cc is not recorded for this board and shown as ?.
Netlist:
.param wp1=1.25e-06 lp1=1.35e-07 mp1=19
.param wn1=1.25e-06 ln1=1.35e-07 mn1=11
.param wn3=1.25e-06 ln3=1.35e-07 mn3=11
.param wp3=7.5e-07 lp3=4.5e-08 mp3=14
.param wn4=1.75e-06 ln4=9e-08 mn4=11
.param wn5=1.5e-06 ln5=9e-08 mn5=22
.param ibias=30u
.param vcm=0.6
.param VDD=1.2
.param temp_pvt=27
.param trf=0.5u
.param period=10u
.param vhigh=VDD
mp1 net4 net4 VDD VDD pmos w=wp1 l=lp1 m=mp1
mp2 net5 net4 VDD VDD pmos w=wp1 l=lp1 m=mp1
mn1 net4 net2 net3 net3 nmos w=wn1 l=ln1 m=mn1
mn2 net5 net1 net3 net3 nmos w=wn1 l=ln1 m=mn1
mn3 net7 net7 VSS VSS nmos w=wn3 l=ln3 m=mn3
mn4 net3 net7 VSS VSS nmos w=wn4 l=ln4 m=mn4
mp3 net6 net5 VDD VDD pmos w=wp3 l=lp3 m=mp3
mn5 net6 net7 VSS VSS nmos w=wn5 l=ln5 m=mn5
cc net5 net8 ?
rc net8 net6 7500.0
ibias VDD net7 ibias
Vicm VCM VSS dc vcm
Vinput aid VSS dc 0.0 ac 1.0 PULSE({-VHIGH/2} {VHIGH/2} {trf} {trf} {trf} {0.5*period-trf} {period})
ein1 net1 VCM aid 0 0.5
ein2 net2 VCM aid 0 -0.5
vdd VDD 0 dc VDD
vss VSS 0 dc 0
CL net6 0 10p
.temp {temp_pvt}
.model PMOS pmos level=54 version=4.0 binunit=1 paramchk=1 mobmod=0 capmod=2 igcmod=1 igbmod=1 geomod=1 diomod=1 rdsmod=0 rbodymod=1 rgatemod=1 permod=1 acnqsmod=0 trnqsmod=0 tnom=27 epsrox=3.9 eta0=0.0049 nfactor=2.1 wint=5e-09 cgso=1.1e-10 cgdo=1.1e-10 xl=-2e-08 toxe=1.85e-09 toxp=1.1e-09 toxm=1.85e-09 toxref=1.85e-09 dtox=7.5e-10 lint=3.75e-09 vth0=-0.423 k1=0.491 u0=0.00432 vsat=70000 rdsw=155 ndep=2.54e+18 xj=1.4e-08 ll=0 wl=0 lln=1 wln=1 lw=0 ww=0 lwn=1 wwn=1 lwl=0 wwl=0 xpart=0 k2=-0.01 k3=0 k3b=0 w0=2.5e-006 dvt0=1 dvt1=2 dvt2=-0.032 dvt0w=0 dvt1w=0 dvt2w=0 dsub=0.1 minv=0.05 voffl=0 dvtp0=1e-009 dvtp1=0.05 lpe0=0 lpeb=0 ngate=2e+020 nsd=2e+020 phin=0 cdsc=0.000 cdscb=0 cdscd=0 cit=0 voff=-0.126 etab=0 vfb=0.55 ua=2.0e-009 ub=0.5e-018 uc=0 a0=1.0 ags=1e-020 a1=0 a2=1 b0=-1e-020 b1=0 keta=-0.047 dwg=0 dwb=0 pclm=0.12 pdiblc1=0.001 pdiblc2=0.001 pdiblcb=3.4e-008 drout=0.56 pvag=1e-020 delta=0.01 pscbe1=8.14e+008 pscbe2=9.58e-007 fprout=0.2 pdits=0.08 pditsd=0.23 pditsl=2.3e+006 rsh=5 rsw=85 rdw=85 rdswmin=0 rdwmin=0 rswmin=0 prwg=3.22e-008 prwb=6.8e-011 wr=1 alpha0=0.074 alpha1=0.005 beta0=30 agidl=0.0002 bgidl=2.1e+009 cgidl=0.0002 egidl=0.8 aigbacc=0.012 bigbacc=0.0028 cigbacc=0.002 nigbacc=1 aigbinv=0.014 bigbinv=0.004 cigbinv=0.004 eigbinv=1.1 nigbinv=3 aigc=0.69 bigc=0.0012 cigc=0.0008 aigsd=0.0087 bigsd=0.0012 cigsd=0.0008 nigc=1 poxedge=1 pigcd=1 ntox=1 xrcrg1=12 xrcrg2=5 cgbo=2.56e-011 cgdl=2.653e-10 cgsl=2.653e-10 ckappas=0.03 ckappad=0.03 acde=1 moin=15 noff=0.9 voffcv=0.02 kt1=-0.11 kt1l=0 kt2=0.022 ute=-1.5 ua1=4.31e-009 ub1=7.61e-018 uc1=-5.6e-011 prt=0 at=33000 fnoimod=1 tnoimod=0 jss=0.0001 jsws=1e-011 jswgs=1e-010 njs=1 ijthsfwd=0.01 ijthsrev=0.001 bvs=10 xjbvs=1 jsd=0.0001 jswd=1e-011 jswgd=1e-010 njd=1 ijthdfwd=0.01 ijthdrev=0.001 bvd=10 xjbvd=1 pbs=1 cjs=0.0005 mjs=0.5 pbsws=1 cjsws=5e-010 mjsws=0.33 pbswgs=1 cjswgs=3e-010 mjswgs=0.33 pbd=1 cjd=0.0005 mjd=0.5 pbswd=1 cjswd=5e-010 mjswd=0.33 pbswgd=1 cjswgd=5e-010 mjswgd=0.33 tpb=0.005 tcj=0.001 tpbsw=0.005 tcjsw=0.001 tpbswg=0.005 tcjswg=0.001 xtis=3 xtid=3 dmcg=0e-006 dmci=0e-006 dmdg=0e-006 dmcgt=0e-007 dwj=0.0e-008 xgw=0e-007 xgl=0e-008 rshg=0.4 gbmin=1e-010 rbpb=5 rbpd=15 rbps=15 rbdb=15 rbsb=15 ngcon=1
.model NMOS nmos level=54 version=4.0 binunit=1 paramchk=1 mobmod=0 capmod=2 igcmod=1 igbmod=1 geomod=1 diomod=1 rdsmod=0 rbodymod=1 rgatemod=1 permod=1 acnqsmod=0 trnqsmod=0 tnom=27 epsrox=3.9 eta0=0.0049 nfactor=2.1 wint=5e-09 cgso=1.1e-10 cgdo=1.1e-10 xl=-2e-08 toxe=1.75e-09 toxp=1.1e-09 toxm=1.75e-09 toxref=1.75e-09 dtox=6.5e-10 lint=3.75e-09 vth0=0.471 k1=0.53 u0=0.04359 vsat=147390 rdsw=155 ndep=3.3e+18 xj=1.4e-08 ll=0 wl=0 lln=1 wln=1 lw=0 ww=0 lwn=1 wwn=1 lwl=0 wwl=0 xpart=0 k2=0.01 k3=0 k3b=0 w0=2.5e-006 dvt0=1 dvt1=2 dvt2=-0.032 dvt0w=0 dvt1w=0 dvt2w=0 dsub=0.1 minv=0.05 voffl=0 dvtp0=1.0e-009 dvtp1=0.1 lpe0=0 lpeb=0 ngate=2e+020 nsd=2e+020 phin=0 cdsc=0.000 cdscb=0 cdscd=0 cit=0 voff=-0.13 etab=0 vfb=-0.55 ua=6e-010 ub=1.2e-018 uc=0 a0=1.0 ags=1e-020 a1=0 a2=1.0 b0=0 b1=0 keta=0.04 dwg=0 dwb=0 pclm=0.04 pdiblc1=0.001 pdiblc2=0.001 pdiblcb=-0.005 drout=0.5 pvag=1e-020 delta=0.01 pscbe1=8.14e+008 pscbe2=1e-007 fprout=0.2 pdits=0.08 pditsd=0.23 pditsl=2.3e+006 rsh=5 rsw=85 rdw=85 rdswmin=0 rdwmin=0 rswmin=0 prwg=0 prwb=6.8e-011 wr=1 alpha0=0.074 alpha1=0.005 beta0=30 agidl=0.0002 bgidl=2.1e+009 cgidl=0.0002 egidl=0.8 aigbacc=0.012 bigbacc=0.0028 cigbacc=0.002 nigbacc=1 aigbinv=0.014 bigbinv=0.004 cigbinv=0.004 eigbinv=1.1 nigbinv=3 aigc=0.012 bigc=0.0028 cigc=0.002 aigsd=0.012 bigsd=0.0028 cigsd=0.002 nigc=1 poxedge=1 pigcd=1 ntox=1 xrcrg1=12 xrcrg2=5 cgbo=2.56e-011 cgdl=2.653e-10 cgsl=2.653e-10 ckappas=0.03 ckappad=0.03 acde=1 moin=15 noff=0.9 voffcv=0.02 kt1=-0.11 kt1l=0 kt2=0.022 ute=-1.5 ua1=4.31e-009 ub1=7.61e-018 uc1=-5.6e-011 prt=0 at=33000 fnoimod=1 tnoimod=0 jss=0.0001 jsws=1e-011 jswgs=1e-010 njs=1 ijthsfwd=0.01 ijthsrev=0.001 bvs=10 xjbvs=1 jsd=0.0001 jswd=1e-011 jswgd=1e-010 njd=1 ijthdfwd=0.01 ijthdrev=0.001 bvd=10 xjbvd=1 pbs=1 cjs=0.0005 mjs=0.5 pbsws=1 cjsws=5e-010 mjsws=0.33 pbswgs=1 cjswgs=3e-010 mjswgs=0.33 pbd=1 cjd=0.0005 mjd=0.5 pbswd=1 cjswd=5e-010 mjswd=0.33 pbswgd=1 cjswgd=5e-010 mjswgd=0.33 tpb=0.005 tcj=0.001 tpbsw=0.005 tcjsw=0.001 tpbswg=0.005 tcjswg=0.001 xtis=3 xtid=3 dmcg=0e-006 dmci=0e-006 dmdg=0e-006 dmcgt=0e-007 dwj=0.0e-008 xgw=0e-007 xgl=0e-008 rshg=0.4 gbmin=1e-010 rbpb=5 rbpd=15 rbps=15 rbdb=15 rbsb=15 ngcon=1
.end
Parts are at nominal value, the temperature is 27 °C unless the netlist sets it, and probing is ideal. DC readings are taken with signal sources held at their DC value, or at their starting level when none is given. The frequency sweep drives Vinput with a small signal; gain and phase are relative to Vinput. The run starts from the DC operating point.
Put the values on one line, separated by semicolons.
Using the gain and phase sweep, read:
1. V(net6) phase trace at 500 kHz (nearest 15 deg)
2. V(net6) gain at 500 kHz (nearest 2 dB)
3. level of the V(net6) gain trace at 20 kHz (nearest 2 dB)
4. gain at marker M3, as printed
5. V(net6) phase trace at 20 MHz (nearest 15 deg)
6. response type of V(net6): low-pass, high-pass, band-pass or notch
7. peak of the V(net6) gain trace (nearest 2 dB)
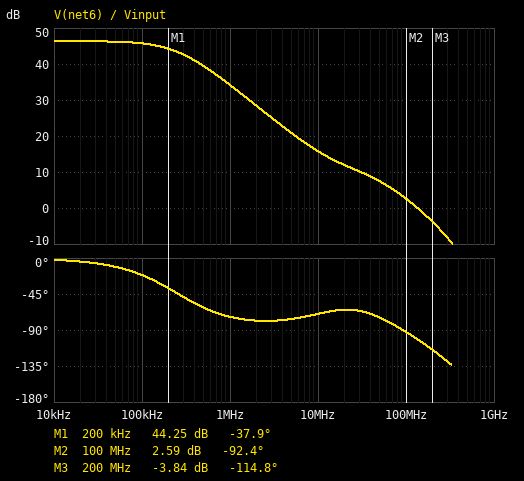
-60 deg; 40 dB; 46 dB; -3.84 dB; -60 deg; low-pass; 46 dB
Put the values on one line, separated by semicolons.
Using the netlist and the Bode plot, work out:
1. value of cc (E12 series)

1.5 pF
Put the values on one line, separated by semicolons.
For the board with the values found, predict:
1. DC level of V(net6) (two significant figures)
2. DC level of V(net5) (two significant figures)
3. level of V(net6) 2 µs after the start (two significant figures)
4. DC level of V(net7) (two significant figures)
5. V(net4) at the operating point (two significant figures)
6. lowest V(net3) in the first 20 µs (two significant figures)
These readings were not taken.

1.0 V; 720 mV; 1.2 V; 400 mV; 720 mV; 4.1 mV
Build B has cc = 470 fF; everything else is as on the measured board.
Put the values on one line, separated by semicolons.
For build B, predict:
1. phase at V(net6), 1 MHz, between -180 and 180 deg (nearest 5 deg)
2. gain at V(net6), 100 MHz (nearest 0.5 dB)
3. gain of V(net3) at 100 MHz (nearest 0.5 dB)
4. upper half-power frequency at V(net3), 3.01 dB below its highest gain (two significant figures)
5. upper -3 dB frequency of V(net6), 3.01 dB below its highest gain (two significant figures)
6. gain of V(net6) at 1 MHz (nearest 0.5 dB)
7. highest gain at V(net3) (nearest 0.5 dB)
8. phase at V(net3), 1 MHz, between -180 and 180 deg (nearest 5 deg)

-55 deg; 3.0 dB; -30.5 dB; 770 kHz; 760 kHz; 42.0 dB; -11.5 dB; 135 deg
